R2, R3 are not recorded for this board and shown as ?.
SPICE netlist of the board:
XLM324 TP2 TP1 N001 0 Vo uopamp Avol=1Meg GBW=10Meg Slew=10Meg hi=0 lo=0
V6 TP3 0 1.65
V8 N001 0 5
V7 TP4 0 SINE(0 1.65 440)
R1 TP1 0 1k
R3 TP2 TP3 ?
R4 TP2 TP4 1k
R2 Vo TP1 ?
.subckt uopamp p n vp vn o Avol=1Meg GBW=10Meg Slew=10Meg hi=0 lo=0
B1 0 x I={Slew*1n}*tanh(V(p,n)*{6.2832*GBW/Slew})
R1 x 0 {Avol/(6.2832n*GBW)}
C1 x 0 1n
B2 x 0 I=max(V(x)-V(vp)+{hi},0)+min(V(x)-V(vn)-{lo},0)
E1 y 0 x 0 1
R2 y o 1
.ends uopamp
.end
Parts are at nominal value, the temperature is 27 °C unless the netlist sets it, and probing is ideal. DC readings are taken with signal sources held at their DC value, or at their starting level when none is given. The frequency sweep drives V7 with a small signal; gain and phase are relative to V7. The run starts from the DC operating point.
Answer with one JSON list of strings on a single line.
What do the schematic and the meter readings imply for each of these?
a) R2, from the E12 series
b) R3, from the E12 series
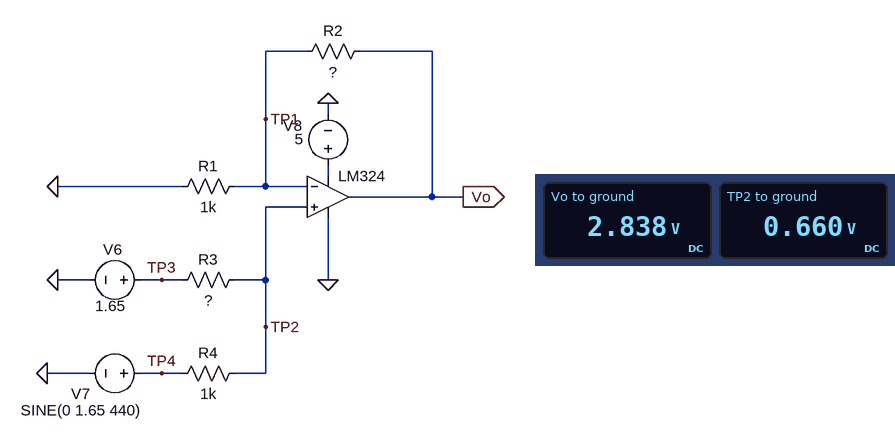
["3.3 kΩ", "1.5 kΩ"]
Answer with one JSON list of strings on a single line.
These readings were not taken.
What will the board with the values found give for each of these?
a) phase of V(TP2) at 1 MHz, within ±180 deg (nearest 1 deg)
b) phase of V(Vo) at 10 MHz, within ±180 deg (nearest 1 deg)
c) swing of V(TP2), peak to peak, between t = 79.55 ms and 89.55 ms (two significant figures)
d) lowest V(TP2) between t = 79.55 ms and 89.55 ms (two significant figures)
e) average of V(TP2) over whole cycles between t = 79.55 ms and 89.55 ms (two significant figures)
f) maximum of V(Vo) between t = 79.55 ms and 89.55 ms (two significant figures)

["0 deg", "-77 deg", "2.0 V", "-330 mV", "660 mV", "5.0 V"]
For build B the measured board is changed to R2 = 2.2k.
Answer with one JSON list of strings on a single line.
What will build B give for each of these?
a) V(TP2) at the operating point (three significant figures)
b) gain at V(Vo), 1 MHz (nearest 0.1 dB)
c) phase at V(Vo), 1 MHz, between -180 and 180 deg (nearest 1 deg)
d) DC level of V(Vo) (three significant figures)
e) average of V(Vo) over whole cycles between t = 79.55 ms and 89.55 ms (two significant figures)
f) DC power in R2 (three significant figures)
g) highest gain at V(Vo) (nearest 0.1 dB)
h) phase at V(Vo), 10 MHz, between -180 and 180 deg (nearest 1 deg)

["660 mV", "5.2 dB", "-18 deg", "2.11 V", "2.3 V", "958 µW", "5.7 dB", "-73 deg"]
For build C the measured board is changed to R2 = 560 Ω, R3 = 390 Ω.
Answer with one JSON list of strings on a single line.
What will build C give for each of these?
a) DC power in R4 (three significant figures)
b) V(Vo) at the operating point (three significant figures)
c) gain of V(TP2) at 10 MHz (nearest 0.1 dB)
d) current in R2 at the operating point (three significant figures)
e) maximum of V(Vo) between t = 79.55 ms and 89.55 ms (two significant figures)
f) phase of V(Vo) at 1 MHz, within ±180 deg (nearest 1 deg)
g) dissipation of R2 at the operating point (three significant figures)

["1.41 mW", "1.85 V", "-11.0 dB", "1.19 mA", "2.6 V", "-9 deg", "789 µW"]
